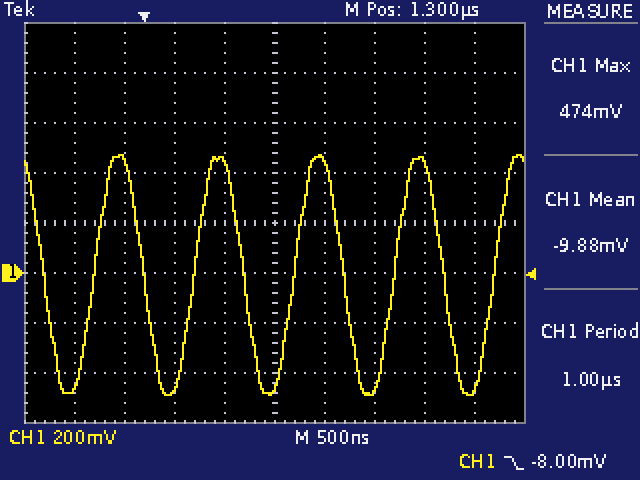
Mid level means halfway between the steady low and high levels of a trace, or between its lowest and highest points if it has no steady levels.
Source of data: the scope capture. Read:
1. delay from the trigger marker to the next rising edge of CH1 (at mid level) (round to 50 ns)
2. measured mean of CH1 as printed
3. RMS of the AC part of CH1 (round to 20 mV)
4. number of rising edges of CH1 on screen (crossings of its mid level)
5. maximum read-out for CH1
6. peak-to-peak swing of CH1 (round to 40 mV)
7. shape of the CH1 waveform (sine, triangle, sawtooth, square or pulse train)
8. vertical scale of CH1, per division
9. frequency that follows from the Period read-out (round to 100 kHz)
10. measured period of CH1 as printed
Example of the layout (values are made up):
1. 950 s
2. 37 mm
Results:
1. 500 ns
2. -9.88 mV
3. 340 mV
4. 5
5. 474 mV
6. 960 mV
7. sine
8. 200 mV
9. 1.0 MHz
10. 1.00 µs
